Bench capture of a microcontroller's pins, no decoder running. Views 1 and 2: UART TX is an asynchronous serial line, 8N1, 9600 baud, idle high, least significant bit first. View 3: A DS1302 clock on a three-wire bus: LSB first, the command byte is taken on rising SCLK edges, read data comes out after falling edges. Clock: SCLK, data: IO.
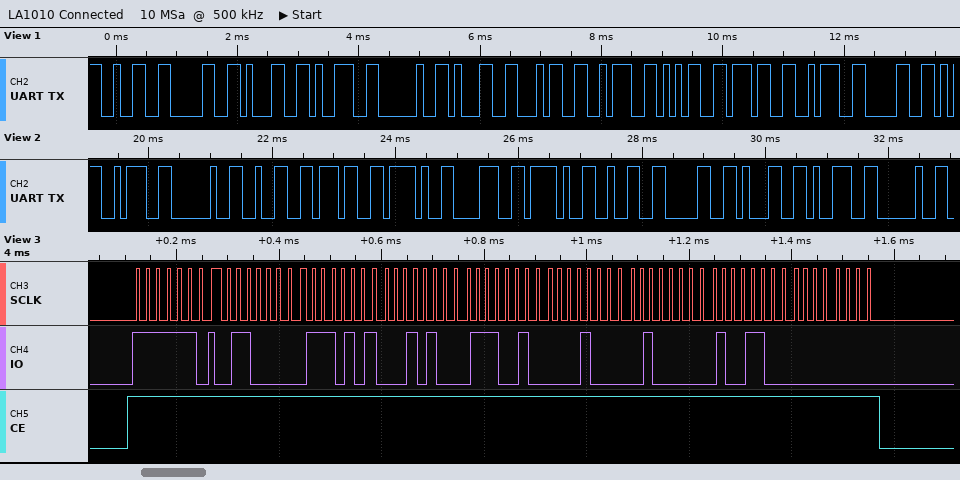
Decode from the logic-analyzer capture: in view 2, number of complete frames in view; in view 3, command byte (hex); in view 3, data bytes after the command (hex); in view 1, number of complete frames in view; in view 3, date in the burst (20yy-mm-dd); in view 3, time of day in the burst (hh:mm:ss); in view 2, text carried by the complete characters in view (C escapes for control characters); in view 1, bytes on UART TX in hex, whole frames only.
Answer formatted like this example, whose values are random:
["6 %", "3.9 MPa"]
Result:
["12", "0xBF", "06 57 14 27 08 02 19 00", "12", "2019-08-27", "14:57:06", "\": 27/8/2019 \"", "32 30 31 39 20 31 34 3A 35 37 3A 30"]
